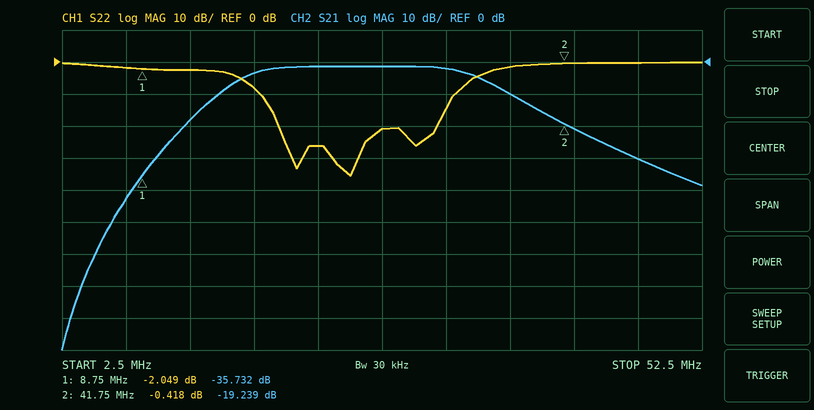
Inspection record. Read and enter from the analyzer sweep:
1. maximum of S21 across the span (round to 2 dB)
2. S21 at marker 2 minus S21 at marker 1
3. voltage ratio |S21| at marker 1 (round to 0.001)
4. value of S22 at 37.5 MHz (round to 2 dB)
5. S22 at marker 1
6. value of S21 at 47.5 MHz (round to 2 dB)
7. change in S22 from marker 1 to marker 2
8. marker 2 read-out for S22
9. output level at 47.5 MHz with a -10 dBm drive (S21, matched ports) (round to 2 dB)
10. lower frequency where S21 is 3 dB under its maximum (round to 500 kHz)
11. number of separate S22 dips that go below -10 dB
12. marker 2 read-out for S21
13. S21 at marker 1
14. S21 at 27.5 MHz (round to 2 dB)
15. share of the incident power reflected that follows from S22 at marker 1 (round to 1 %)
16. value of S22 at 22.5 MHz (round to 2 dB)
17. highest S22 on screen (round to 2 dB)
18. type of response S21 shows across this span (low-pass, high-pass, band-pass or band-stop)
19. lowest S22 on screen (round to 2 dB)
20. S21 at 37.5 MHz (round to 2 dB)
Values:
-2 dB
16.493 dB
0.016
-2 dB
-2.049 dB
-30 dB
1.631 dB
-0.418 dB
-40 dBm
17.0 MHz
3
-19.239 dB
-35.732 dB
-2 dB
62 %
-26 dB
0 dB
band-pass
-36 dB
-10 dB
